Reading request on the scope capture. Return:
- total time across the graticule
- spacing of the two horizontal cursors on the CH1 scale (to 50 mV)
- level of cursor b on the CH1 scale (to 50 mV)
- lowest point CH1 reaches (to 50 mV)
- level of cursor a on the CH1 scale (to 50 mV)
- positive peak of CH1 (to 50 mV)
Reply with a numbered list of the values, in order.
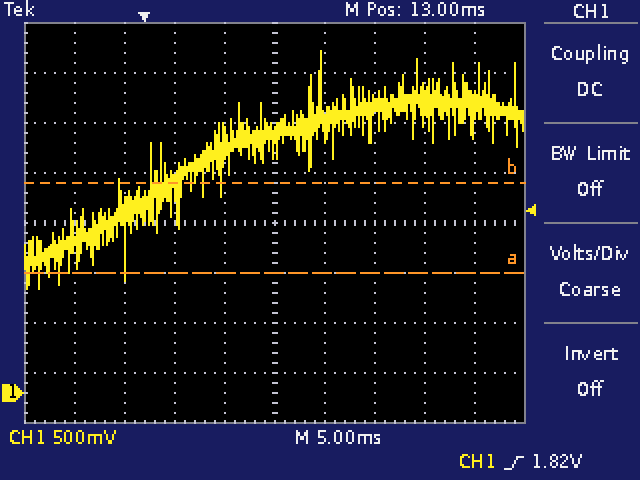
1. 50 ms
2. 900 mV
3. 2.10 V
4. 1.05 V
5. 1.20 V
6. 3.40 V
